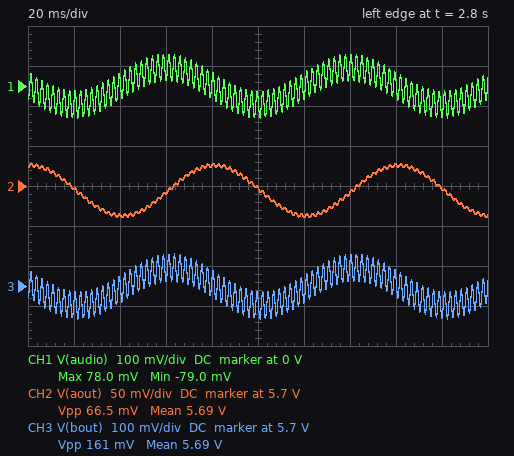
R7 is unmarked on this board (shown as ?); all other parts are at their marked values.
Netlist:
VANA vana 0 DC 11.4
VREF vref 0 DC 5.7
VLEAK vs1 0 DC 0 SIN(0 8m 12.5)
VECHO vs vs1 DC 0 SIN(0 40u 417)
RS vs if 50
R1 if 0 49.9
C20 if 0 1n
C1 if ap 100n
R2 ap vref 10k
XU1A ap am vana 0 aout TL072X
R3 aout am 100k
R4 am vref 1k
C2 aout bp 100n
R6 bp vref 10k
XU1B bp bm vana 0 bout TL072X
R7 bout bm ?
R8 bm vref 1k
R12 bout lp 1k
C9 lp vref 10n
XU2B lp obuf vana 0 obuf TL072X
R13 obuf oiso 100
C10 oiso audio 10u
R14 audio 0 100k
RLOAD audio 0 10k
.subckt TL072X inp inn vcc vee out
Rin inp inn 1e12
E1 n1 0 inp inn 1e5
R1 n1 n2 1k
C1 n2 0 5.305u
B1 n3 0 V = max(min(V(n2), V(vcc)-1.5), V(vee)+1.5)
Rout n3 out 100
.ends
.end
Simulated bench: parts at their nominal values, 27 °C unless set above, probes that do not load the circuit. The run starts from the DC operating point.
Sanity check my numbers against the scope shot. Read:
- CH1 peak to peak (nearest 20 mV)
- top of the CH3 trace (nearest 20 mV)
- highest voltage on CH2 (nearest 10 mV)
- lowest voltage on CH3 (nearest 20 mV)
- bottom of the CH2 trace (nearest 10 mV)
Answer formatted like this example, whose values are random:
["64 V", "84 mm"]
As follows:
["160 mV", "5.78 V", "5.73 V", "5.62 V", "5.66 V"]
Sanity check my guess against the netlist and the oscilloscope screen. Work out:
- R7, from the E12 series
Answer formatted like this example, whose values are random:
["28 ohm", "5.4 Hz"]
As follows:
["18 kΩ"]
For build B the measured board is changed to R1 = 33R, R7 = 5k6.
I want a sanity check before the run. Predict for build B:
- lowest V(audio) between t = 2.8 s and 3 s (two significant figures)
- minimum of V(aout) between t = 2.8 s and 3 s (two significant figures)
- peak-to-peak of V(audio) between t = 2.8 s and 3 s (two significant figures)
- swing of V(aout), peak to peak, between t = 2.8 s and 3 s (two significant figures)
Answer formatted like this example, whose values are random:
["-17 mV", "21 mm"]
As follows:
["-22 mV", "5.7 V", "44 mV", "53 mV"]
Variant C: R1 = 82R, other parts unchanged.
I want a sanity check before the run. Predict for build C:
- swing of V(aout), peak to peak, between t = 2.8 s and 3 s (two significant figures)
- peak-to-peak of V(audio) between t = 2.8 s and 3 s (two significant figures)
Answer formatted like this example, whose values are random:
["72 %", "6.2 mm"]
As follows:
["83 mV", "200 mV"]
